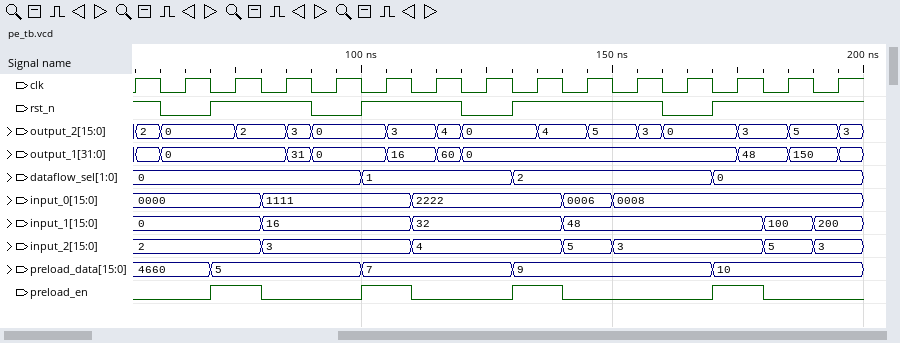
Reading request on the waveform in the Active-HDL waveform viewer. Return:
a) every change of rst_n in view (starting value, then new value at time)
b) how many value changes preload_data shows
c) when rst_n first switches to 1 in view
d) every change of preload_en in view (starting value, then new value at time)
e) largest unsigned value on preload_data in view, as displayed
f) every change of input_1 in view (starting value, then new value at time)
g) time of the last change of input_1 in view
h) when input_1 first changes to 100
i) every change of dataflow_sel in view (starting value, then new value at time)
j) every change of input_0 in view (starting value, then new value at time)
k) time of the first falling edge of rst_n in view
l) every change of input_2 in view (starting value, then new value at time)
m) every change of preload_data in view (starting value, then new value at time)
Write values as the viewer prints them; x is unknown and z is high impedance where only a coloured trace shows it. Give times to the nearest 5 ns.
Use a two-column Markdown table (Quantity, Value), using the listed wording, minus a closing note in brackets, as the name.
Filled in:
| Quantity | Value |
|---|---|
| every change of rst_n in view | 1, 0 at 60 ns, 1 at 70 ns, 0 at 90 ns, 1 at 100 ns, 0 at 120 ns, 1 at 130 ns, 0 at 160 ns, 1 at 170 ns |
| how many value changes preload_data shows | 4 |
| when rst_n first switches to 1 in view | 70 ns |
| every change of preload_en in view | 0, 1 at 70 ns, 0 at 80 ns, 1 at 100 ns, 0 at 110 ns, 1 at 130 ns, 0 at 140 ns, 1 at 170 ns, 0 at 180 ns |
| largest unsigned value on preload_data in view, as displayed | 4660 |
| every change of input_1 in view | 0, 16 at 80 ns, 32 at 110 ns, 48 at 140 ns, 100 at 180 ns, 200 at 190 ns |
| time of the last change of input_1 in view | 190 ns |
| when input_1 first changes to 100 | 180 ns |
| every change of dataflow_sel in view | 0, 1 at 100 ns, 2 at 130 ns, 0 at 170 ns |
| every change of input_0 in view | 0000, 1111 at 80 ns, 2222 at 110 ns, 0006 at 140 ns, 0008 at 150 ns |
| time of the first falling edge of rst_n in view | 60 ns |
| every change of input_2 in view | 2, 3 at 80 ns, 4 at 110 ns, 5 at 140 ns, 3 at 150 ns, 5 at 180 ns, 3 at 190 ns |
| every change of preload_data in view | 4660, 5 at 70 ns, 7 at 100 ns, 9 at 130 ns, 10 at 170 ns |
